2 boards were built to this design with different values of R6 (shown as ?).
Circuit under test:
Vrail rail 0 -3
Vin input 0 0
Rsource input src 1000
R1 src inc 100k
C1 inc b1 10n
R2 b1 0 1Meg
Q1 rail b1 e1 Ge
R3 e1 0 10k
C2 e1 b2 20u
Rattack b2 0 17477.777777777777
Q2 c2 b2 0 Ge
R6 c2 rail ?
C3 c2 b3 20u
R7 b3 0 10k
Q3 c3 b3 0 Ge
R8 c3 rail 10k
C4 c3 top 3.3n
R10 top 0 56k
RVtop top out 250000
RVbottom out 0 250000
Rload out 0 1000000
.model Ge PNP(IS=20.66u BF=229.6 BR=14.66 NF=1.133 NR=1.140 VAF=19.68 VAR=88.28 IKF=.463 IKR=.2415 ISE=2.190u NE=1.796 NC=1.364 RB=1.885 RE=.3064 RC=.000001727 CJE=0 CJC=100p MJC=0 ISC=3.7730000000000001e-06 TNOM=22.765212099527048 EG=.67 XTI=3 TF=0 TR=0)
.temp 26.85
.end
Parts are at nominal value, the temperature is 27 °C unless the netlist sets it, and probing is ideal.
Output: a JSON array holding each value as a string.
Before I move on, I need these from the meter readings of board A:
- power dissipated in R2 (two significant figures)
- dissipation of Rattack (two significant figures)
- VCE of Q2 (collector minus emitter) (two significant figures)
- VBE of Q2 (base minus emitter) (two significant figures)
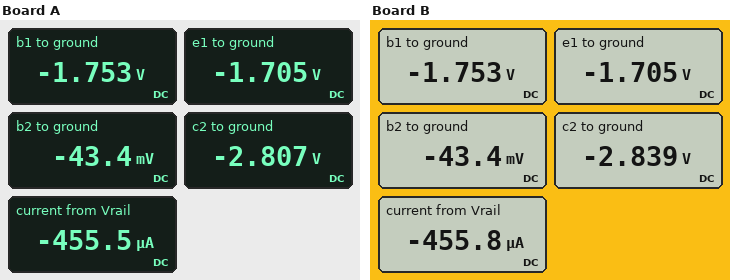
["3.1 µW", "110 nW", "-2.8 V", "-43 mV"]
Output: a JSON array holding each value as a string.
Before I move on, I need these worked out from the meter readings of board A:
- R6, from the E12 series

["1.2 kΩ"]
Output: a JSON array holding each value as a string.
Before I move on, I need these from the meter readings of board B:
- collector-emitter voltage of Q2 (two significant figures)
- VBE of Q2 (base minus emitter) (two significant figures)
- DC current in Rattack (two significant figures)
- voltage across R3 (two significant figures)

["-2.8 V", "-43 mV", "2.5 µA", "1.7 V"]
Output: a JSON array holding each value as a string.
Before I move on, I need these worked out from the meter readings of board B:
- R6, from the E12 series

["1 kΩ"]
